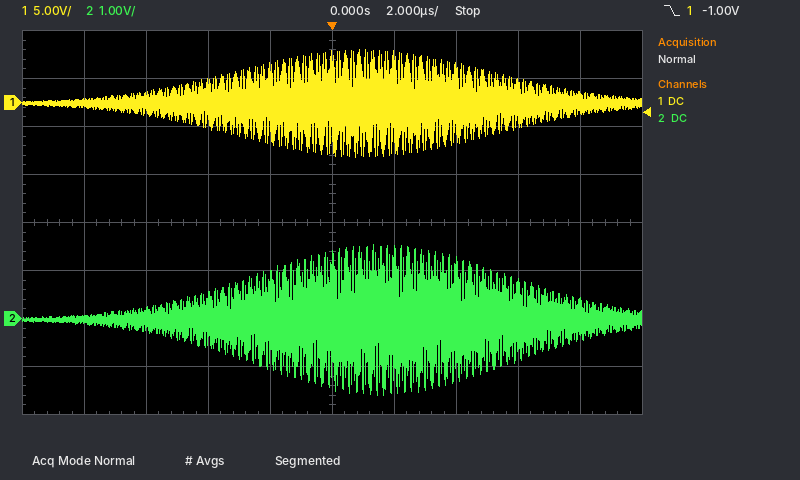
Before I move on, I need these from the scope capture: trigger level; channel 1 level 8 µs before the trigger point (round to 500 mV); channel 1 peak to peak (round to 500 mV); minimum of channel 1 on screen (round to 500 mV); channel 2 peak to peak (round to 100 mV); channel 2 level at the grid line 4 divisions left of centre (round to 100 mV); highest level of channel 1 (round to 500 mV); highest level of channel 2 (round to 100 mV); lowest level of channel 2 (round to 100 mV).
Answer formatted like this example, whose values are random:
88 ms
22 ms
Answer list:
-1.00 V
0.0 V
11.0 V
-5.5 V
3.1 V
0.0 V
5.5 V
1.5 V
-1.6 V
